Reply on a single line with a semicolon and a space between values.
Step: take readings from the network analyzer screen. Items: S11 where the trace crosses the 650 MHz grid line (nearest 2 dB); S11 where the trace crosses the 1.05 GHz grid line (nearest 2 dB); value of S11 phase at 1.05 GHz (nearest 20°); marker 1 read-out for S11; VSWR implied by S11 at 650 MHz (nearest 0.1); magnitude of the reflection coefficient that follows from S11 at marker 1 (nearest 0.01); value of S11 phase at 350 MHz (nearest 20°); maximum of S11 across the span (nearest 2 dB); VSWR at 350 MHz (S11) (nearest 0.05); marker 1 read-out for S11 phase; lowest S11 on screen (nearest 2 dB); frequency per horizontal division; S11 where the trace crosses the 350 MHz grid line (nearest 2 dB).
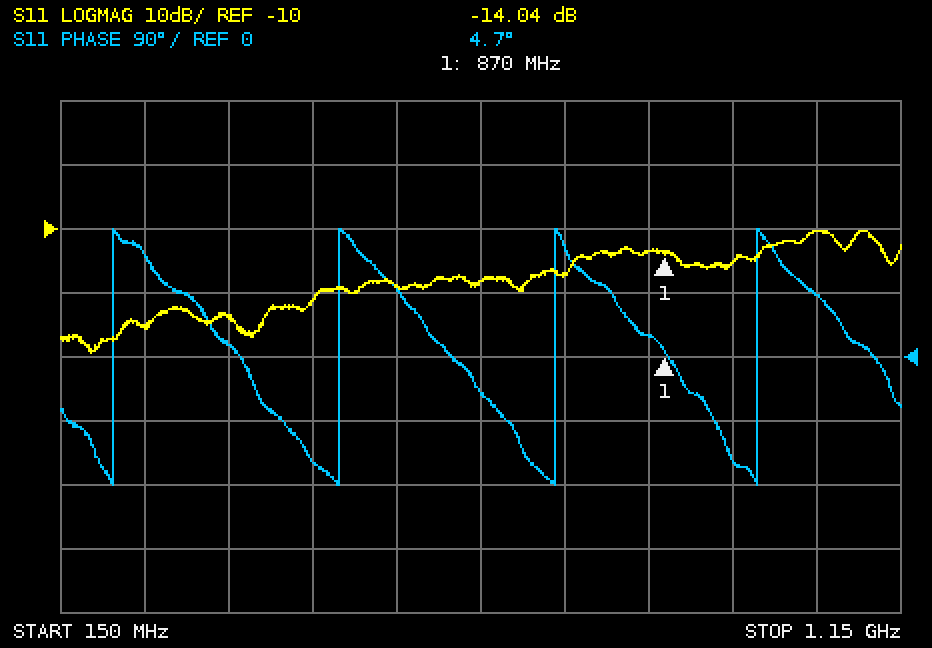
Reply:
-18 dB; -10 dB; 80°; -14.04 dB; 1.3; 0.20; 20°; -10 dB; 1.15; 4.7°; -30 dB; 100 MHz; -24 dB
